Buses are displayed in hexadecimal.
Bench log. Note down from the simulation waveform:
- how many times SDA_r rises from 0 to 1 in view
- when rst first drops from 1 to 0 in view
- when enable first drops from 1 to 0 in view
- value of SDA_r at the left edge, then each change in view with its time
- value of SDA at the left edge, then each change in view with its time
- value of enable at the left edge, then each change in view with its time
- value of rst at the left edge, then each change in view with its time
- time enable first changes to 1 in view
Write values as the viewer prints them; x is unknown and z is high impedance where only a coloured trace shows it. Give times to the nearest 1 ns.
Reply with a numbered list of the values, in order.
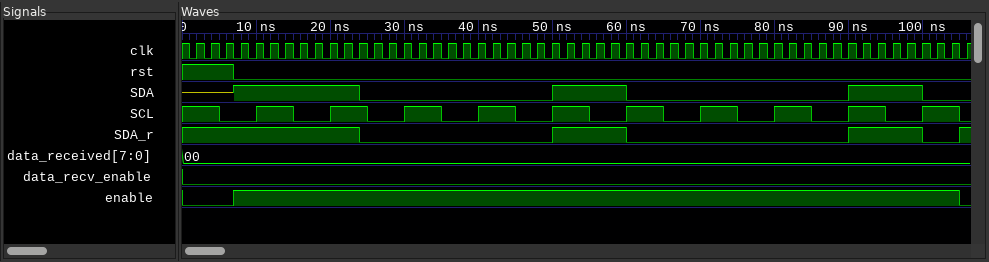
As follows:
1. 3
2. 7 ns
3. 105 ns
4. 1, 0 at 24 ns, 1 at 50 ns, 0 at 60 ns, 1 at 90 ns, 0 at 100 ns, 1 at 105 ns
5. z, 1 at 7 ns, 0 at 24 ns, 1 at 50 ns, 0 at 60 ns, 1 at 90 ns, 0 at 100 ns
6. 0, 1 at 7 ns, 0 at 105 ns
7. 1, 0 at 7 ns
8. 7 ns
